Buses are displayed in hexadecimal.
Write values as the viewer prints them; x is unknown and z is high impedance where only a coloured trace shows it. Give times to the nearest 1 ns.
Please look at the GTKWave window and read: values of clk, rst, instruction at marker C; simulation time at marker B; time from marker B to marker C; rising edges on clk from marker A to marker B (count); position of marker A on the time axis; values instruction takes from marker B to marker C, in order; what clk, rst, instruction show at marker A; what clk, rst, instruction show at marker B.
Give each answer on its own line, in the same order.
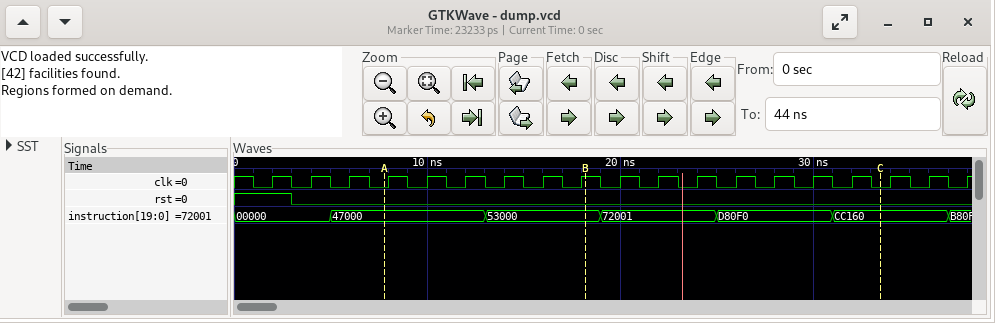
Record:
clk=0, rst=0, instruction=CC160
18 ns
15 ns
6
8 ns
53000, 72001, D80F0, CC160
clk=0, rst=0, instruction=47000
clk=1, rst=0, instruction=53000
